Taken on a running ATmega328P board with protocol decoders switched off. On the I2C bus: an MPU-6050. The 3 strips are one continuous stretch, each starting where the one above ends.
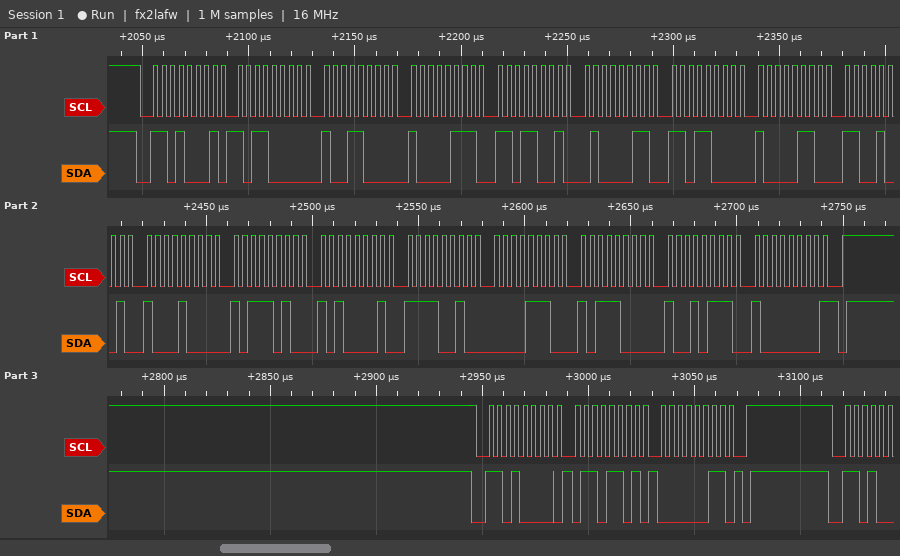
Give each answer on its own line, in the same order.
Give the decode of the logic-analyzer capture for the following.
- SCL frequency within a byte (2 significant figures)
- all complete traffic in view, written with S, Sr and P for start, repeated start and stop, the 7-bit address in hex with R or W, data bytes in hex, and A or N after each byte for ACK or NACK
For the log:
250 kHz
S 68R A B0 A 98 A 87 A D9 A 43 A D8 A 86 A C9 A 88 A BA A A1 A F2 A 0E A B8 A 97 A 80 N P S 68W A 6D A 03 A P
